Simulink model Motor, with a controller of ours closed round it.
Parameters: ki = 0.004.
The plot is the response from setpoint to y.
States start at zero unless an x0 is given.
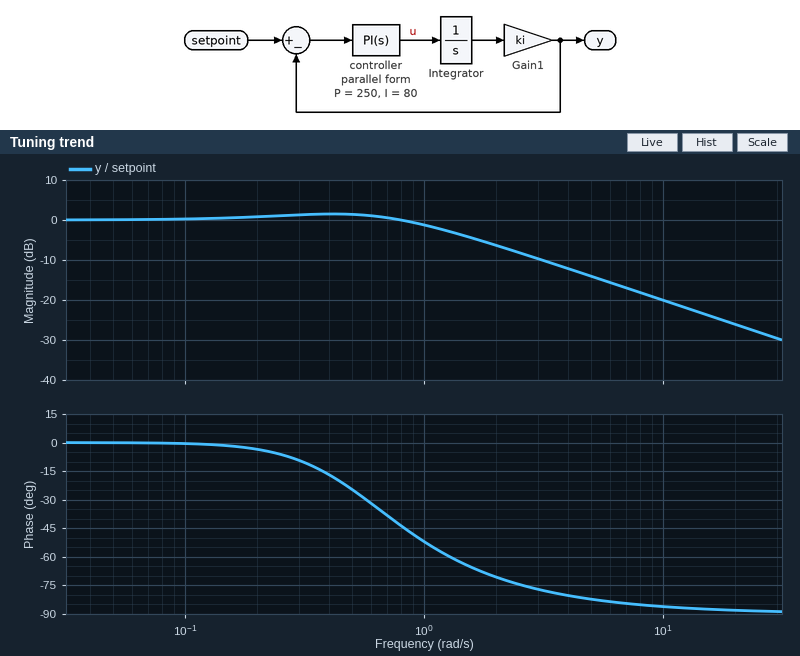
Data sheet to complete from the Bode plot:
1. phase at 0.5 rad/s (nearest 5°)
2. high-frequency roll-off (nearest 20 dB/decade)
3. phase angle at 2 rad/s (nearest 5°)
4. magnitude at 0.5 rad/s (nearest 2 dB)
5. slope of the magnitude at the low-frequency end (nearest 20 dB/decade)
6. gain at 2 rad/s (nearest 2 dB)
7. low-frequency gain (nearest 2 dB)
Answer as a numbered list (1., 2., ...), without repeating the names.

1. -25°
2. -20 dB/decade
3. -70°
4. 2 dB
5. 0 dB/decade
6. -6 dB
7. 0 dB
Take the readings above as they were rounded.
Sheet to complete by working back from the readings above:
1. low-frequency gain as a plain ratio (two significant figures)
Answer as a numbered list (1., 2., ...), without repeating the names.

1. 1.0
